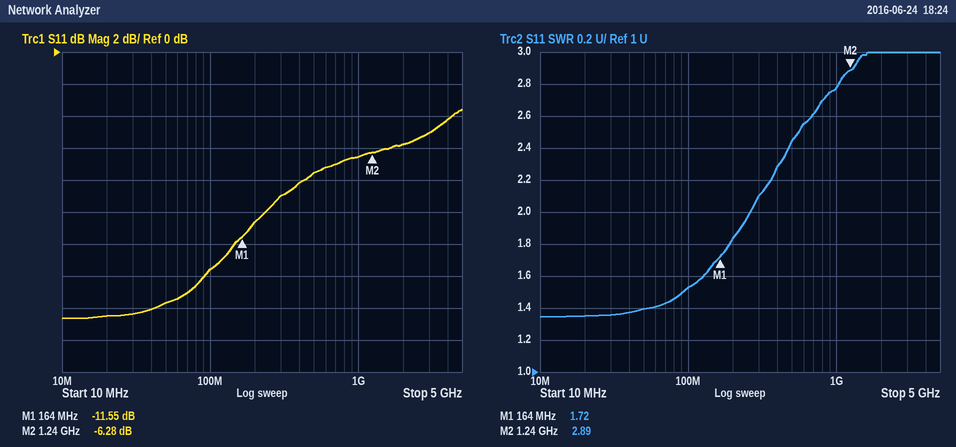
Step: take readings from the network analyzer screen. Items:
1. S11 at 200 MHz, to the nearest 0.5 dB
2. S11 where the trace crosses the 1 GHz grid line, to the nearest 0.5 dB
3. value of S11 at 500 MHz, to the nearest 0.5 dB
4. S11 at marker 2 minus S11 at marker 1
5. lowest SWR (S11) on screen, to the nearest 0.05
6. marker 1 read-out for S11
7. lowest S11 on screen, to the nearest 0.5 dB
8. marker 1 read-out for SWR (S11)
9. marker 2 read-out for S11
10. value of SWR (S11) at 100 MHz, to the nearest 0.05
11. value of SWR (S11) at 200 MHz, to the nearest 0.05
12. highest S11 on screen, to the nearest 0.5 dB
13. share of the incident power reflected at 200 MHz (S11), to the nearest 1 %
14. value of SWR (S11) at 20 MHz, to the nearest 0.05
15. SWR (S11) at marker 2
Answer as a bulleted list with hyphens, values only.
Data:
- -10.5 dB
- -6.5 dB
- -7.5 dB
- 5.27 dB
- 1.35
- -11.55 dB
- -16.5 dB
- 1.72
- -6.28 dB
- 1.55
- 1.85
- -3.5 dB
- 9 %
- 1.35
- 2.89
